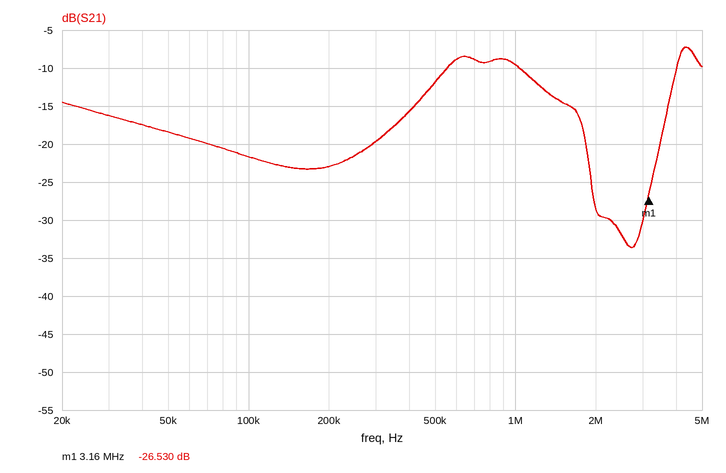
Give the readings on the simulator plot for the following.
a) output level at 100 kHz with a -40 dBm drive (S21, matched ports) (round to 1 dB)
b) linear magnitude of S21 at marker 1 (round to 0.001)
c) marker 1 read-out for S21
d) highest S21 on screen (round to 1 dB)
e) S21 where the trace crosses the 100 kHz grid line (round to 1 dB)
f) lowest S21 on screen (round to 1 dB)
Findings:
-62 dBm
0.047
-26.530 dB
-7 dB
-22 dB
-34 dB
